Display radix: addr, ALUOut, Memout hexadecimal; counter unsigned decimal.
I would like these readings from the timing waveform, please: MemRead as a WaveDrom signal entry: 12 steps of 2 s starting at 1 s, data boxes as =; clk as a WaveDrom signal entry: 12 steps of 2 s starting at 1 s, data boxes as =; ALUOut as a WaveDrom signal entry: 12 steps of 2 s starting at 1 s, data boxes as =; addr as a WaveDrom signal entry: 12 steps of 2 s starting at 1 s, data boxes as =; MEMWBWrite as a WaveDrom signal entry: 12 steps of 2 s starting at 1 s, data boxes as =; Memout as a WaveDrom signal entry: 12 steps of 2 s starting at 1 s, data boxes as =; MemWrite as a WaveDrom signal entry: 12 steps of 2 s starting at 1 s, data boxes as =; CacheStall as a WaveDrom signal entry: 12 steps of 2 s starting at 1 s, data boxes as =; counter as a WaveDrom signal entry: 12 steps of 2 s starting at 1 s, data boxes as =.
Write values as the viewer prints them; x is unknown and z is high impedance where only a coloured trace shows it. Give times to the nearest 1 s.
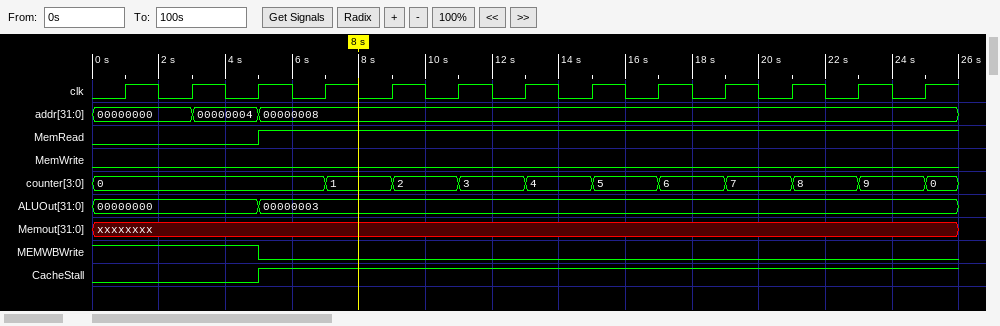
{name: 'MemRead', wave: '0.1.........'}
{name: 'clk', wave: 'p...........'}
{name: 'ALUOut', wave: '=.=.........', data: '00000000 00000003'}
{name: 'addr', wave: '===.........', data: '00000000 00000004 00000008'}
{name: 'MEMWBWrite', wave: '1.0.........'}
{name: 'Memout', wave: 'x...........'}
{name: 'MemWrite', wave: '0...........'}
{name: 'CacheStall', wave: '0.1.........'}
{name: 'counter', wave: '=..=========', data: '0 1 2 3 4 5 6 7 8 9'}
